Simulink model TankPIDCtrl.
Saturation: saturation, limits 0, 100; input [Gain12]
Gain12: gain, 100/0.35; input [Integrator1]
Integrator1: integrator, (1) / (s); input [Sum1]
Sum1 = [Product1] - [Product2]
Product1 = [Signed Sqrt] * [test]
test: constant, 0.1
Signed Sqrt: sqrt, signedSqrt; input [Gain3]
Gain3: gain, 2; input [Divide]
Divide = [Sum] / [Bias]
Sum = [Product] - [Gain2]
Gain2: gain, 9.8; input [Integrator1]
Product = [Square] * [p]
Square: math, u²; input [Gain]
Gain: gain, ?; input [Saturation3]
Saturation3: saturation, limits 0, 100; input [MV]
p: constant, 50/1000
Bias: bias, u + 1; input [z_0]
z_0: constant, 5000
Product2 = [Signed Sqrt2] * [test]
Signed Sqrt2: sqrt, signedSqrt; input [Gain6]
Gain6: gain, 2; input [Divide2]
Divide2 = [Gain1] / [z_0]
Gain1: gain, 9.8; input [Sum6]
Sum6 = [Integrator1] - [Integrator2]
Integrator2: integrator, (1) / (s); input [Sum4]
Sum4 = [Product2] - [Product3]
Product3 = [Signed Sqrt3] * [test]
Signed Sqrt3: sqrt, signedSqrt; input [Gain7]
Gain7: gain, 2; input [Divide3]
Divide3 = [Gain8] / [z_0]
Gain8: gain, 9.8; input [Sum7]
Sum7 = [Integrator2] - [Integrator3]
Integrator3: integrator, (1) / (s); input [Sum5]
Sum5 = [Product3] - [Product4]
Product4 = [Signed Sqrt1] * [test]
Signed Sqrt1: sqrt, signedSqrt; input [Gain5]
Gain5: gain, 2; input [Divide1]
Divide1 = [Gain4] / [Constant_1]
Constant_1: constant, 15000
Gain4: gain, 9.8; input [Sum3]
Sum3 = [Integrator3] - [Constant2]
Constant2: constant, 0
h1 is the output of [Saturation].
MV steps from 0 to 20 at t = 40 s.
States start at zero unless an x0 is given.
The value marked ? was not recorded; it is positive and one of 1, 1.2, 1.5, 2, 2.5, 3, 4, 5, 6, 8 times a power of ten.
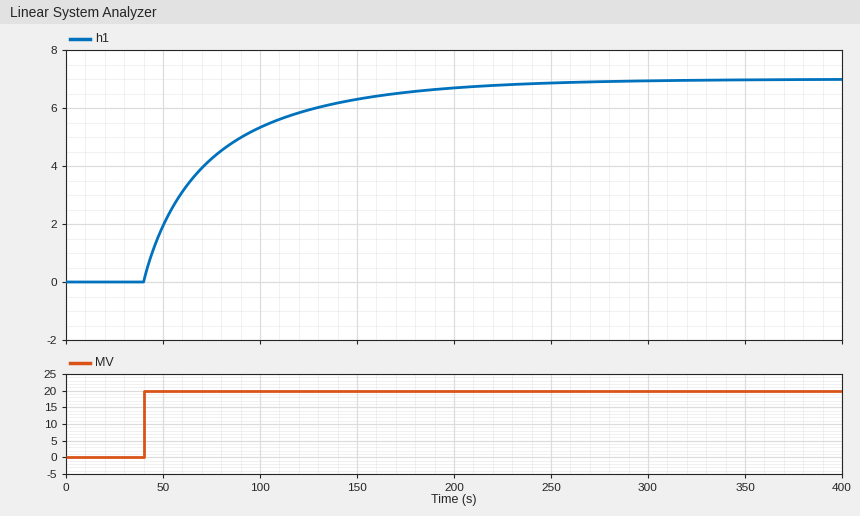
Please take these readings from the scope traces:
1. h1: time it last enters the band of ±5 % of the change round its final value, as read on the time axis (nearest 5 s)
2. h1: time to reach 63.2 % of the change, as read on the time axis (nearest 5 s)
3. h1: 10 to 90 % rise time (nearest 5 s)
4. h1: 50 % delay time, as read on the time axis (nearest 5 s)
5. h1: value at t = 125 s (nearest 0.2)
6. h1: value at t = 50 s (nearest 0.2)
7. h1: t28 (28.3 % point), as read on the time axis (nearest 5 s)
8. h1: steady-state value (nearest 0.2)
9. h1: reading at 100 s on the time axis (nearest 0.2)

190 s
80 s
105 s
65 s
6.0
2.0
50 s
7.0
5.4
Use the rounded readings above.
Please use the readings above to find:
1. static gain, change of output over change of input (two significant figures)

0.35
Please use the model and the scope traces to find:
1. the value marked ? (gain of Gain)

0.12
